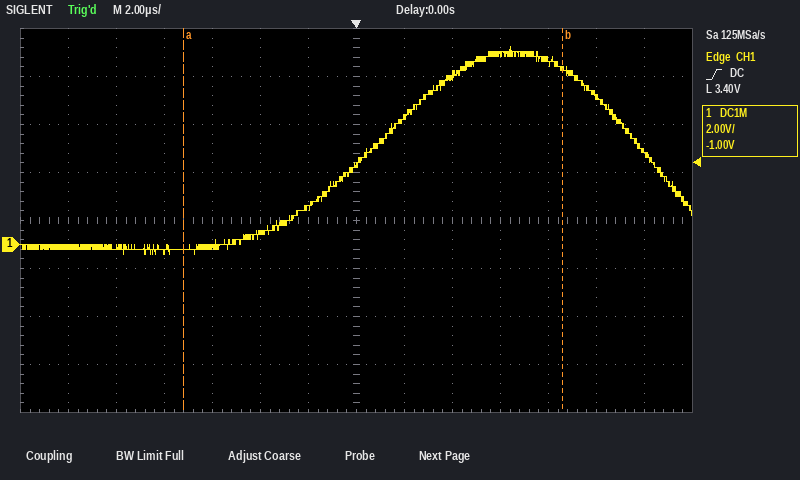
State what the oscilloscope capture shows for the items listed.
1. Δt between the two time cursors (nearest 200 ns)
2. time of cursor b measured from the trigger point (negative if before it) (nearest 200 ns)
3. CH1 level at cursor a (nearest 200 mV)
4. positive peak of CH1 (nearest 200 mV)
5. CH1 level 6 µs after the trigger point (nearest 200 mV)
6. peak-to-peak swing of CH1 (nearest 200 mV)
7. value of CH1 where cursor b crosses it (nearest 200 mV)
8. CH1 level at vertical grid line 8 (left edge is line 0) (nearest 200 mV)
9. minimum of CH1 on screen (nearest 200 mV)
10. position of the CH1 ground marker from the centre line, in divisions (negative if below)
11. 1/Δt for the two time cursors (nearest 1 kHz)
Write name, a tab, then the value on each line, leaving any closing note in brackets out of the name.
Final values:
Δt between the two time cursors	15.8 µs
time of cursor b measured from the trigger point (negative if before it)	+8.6 µs
CH1 level at cursor a	-200 mV
positive peak of CH1	8.2 V
CH1 level 6 µs after the trigger point	8.0 V
peak-to-peak swing of CH1	8.6 V
value of CH1 where cursor b crosses it	7.4 V
CH1 level at vertical grid line 8 (left edge is line 0)	5.4 V
minimum of CH1 on screen	-400 mV
position of the CH1 ground marker from the centre line, in divisions	-0.5 div
1/Δt for the two time cursors	63 kHz
